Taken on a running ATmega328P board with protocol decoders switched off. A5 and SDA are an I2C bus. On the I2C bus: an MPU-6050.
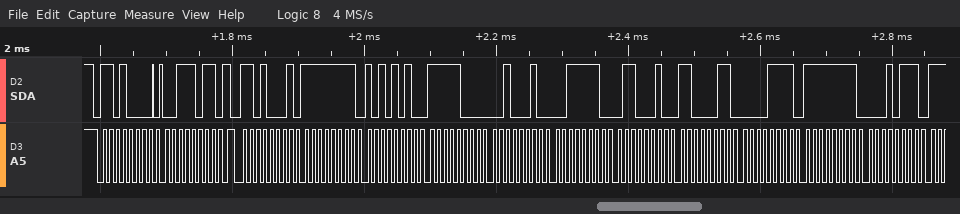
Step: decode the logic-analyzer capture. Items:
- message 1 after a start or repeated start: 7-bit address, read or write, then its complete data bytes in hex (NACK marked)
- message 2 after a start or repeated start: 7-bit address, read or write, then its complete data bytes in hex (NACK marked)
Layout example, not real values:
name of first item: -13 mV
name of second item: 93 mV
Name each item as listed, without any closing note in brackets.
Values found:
message 1 after a start or repeated start: 7-bit address, read or write, then its complete data bytes in hex: 0x68 write: 3B
message 2 after a start or repeated start: 7-bit address, read or write, then its complete data bytes in hex: 0x68 read: FF AA F8 22 3E 62 C3 0F FF 17
